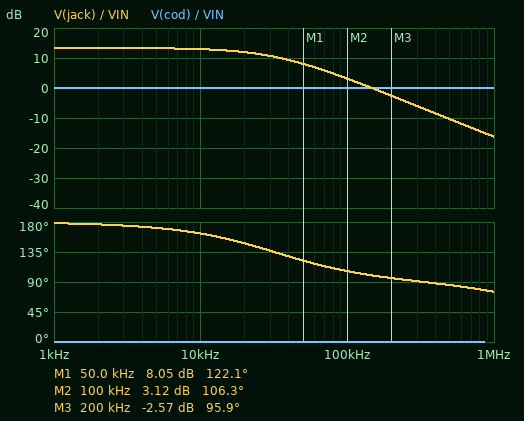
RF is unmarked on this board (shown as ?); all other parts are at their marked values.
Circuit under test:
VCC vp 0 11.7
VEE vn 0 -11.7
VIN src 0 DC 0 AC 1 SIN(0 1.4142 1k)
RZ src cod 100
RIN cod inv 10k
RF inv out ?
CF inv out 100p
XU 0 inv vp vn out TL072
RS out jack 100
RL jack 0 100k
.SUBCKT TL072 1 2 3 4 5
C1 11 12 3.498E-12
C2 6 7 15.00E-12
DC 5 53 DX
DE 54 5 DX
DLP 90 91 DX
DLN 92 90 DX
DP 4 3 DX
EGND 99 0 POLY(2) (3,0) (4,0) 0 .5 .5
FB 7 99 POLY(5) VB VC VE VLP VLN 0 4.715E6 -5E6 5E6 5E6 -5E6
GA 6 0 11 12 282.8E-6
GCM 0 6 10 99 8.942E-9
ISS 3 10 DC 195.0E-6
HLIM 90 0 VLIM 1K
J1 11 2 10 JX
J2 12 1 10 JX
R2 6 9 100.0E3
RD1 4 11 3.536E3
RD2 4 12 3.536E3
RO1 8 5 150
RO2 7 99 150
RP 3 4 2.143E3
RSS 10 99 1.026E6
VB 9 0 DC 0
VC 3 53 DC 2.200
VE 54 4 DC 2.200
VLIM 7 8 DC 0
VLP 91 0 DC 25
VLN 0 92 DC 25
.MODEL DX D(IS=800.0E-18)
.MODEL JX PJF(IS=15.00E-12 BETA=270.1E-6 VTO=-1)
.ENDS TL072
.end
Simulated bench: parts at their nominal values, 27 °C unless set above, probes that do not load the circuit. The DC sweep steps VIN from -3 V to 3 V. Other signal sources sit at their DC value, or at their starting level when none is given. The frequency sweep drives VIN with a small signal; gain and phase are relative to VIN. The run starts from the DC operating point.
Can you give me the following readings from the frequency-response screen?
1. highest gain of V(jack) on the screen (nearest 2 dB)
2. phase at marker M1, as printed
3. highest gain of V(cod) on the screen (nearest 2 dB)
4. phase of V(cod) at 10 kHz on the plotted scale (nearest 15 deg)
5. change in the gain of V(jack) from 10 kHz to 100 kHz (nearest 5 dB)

14 dB
122.1 deg
0 dB
0 deg
-10 dB
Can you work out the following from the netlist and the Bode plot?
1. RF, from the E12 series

47 kΩ
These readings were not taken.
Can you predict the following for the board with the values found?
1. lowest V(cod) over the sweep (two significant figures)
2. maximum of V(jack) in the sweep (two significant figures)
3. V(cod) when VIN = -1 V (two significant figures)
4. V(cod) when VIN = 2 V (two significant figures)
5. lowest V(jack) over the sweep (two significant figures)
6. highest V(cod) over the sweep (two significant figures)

-3.0 V
10 V
-990 mV
2.0 V
-10 V
3.0 V
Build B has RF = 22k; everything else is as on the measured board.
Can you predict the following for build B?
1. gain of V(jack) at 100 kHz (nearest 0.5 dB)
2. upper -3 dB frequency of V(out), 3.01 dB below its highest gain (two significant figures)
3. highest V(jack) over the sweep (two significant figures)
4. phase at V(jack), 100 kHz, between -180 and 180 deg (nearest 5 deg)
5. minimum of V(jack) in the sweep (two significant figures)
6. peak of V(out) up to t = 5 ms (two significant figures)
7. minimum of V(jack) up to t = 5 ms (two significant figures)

2.0 dB
69 kHz
6.5 V
125 deg
-6.5 V
3.1 V
-3.1 V
